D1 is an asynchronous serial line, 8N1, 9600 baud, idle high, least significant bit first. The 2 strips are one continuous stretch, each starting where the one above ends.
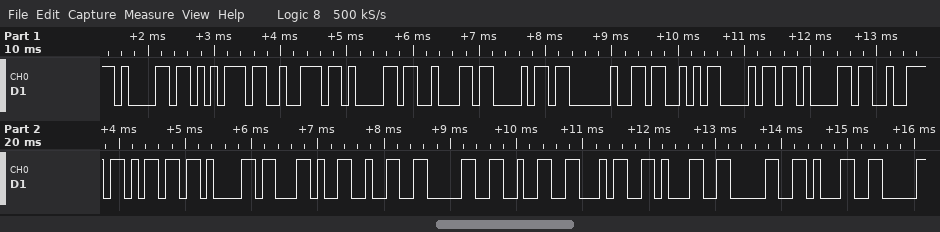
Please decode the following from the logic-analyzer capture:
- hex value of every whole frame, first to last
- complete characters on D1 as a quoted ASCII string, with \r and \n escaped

61 75 72 61 62 68 20 53 68 61 72 6D 61 2C 32 30 32 34 31 30 31
"aurabh Sharma,2024101"
